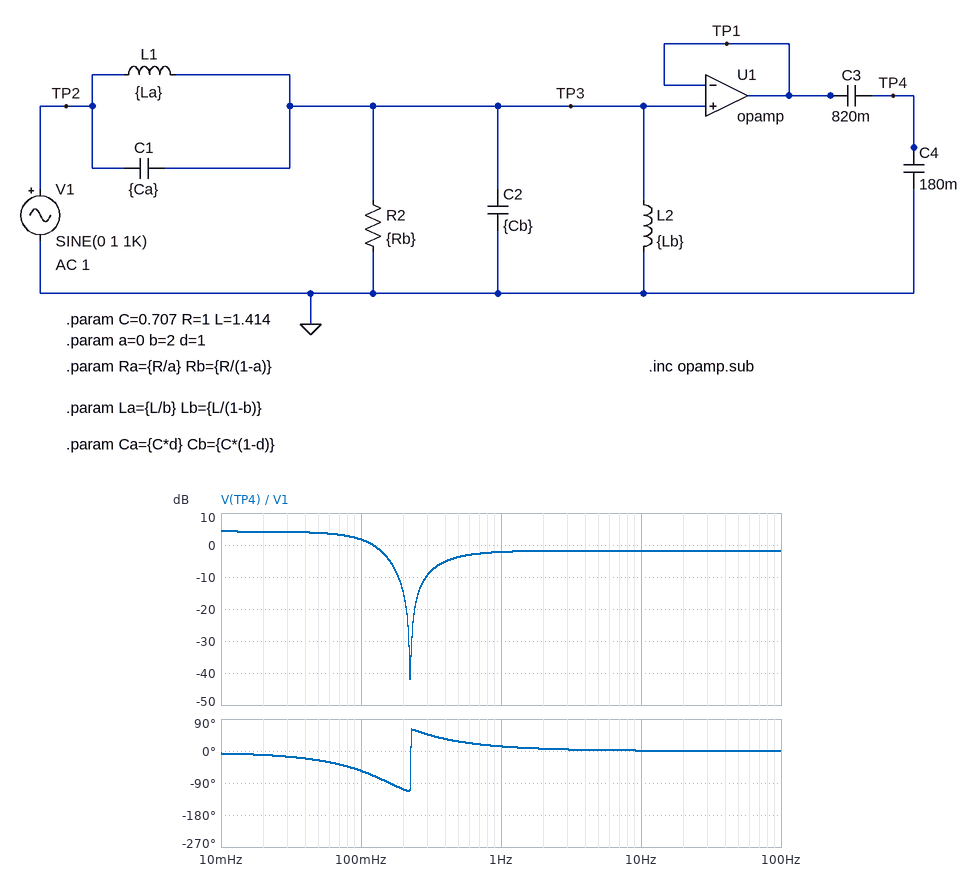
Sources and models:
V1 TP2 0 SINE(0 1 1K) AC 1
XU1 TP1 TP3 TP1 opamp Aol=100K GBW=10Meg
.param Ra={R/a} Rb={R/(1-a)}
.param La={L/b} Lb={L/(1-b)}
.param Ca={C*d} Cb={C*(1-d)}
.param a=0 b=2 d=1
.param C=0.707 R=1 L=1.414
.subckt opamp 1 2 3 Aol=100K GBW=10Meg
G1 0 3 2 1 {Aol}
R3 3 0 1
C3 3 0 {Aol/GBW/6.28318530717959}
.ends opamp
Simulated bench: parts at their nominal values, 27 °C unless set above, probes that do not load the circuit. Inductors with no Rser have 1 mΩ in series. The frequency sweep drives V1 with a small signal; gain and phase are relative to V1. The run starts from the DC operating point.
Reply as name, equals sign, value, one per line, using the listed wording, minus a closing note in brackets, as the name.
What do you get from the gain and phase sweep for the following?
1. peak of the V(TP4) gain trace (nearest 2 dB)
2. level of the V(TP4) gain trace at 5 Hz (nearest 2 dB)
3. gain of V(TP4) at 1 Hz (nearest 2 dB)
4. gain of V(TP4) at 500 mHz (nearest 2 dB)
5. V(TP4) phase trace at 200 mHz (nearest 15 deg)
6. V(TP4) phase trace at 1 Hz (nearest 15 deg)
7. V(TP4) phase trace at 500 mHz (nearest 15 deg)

peak of the V(TP4) gain trace = 4 dB
level of the V(TP4) gain trace at 5 Hz = -2 dB
gain of V(TP4) at 1 Hz = -2 dB
gain of V(TP4) at 500 mHz = -4 dB
V(TP4) phase trace at 200 mHz = -105 deg
V(TP4) phase trace at 1 Hz = 15 deg
V(TP4) phase trace at 500 mHz = 30 deg
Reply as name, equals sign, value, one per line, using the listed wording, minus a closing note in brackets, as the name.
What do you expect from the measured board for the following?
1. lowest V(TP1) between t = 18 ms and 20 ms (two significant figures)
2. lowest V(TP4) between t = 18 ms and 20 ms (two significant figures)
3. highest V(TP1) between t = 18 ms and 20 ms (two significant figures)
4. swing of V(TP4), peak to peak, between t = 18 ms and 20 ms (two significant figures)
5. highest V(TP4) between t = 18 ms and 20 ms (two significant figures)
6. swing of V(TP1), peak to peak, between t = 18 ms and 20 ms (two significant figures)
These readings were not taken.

lowest V(TP1) between t = 18 ms and 20 ms = -1.0 V
lowest V(TP4) between t = 18 ms and 20 ms = -820 mV
highest V(TP1) between t = 18 ms and 20 ms = 1.0 V
swing of V(TP4), peak to peak, between t = 18 ms and 20 ms = 1.6 V
highest V(TP4) between t = 18 ms and 20 ms = 820 mV
swing of V(TP1), peak to peak, between t = 18 ms and 20 ms = 2.0 V
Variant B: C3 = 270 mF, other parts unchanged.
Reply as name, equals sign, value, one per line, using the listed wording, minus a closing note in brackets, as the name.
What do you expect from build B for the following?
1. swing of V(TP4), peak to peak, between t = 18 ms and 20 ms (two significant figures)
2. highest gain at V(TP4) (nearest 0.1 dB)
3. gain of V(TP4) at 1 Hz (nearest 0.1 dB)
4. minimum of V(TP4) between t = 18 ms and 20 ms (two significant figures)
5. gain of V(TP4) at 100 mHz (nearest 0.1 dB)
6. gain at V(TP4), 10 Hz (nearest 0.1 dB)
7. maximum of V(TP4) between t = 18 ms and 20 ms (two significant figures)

swing of V(TP4), peak to peak, between t = 18 ms and 20 ms = 1.2 V
highest gain at V(TP4) = 1.5 dB
gain of V(TP4) at 1 Hz = -4.9 dB
minimum of V(TP4) between t = 18 ms and 20 ms = -600 mV
gain of V(TP4) at 100 mHz = -1.0 dB
gain at V(TP4), 10 Hz = -4.4 dB
maximum of V(TP4) between t = 18 ms and 20 ms = 600 mV
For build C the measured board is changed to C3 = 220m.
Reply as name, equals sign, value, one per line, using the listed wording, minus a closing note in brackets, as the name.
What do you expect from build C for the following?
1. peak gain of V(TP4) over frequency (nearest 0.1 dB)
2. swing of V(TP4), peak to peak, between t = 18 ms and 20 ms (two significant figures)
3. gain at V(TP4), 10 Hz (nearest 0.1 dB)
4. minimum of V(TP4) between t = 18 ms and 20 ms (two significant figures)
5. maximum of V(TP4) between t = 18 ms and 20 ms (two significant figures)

peak gain of V(TP4) over frequency = 0.8 dB
swing of V(TP4), peak to peak, between t = 18 ms and 20 ms = 1.1 V
gain at V(TP4), 10 Hz = -5.2 dB
minimum of V(TP4) between t = 18 ms and 20 ms = -550 mV
maximum of V(TP4) between t = 18 ms and 20 ms = 550 mV
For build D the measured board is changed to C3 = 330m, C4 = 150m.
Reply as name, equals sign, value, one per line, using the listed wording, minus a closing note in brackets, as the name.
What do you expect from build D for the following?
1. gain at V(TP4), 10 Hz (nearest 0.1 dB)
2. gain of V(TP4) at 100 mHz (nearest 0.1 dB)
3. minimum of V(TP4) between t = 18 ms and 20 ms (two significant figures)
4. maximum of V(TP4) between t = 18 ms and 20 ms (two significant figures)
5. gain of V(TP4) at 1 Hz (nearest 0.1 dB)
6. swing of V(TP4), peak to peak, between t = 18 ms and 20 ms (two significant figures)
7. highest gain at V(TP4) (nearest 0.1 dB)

gain at V(TP4), 10 Hz = -3.3 dB
gain of V(TP4) at 100 mHz = 0.2 dB
minimum of V(TP4) between t = 18 ms and 20 ms = -690 mV
maximum of V(TP4) between t = 18 ms and 20 ms = 690 mV
gain of V(TP4) at 1 Hz = -3.7 dB
swing of V(TP4), peak to peak, between t = 18 ms and 20 ms = 1.4 V
highest gain at V(TP4) = 2.7 dB
